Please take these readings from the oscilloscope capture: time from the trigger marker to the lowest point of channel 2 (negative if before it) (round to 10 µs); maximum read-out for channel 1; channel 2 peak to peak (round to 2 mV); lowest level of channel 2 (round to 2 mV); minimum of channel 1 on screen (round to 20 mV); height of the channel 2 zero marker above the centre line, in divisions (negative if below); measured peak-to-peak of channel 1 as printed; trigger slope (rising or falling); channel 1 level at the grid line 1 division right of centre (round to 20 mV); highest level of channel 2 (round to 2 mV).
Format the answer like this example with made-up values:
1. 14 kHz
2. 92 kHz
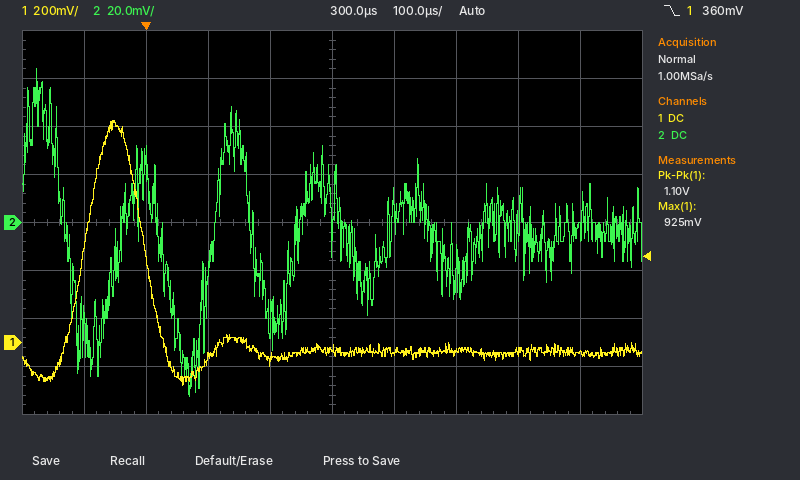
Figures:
1. +70 µs
2. 925 mV
3. 136 mV
4. -72 mV
5. -180 mV
6. 0.0 div
7. 1.10 V
8. falling
9. -40 mV
10. 64 mV
